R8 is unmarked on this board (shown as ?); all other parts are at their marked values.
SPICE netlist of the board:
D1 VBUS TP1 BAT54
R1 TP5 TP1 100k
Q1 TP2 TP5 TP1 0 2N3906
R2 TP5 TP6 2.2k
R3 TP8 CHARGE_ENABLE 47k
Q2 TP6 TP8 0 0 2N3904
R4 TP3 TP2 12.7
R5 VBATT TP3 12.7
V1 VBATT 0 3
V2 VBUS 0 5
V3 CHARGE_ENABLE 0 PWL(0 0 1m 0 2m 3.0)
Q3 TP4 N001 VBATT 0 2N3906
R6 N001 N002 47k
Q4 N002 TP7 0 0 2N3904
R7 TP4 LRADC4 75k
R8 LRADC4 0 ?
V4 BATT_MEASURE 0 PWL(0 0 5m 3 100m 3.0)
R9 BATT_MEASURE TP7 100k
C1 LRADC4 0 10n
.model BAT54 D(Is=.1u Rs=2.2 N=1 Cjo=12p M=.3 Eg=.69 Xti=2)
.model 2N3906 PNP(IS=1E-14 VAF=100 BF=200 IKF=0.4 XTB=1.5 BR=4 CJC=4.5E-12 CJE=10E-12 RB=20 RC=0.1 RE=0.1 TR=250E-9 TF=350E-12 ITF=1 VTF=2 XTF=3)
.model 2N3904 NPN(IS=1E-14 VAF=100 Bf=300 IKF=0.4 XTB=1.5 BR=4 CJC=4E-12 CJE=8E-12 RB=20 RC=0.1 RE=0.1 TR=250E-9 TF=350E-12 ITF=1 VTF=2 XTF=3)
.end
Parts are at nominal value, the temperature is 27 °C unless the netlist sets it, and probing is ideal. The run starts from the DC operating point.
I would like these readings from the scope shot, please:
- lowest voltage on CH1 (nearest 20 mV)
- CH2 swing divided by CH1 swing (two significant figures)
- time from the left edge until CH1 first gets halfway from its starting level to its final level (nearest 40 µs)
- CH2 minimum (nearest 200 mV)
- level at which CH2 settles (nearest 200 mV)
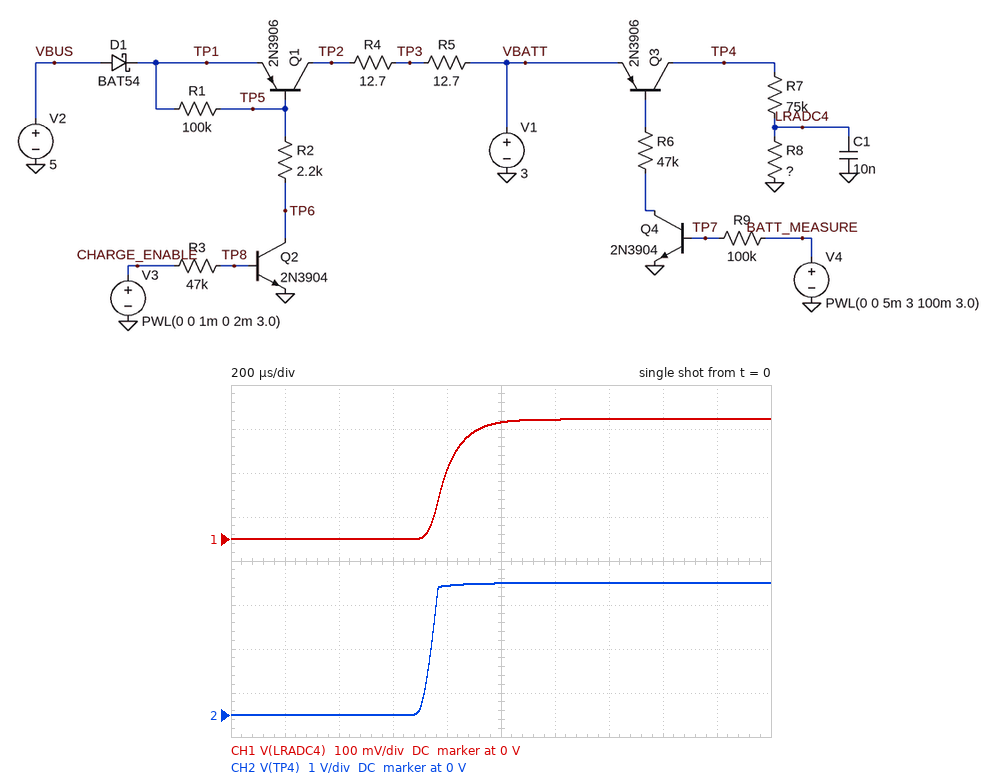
0 V
11
800 µs
0 V
3.0 V
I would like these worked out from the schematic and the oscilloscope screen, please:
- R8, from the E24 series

7.5 kΩ
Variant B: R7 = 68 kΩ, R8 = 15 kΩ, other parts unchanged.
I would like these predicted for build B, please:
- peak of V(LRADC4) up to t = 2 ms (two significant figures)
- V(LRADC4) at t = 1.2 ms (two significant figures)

540 mV
530 mV
